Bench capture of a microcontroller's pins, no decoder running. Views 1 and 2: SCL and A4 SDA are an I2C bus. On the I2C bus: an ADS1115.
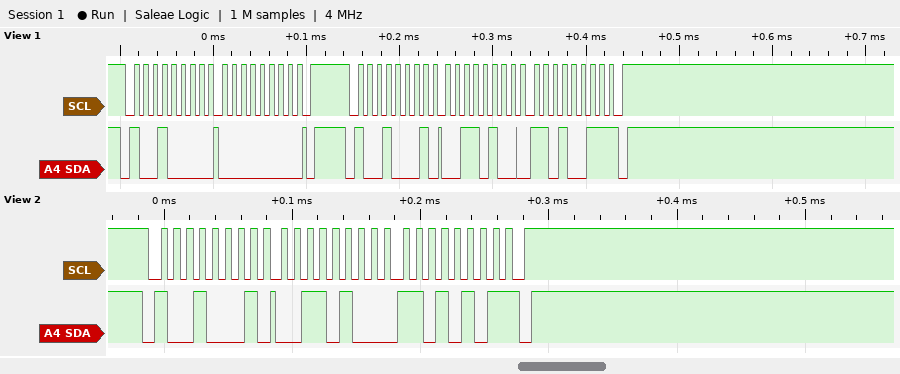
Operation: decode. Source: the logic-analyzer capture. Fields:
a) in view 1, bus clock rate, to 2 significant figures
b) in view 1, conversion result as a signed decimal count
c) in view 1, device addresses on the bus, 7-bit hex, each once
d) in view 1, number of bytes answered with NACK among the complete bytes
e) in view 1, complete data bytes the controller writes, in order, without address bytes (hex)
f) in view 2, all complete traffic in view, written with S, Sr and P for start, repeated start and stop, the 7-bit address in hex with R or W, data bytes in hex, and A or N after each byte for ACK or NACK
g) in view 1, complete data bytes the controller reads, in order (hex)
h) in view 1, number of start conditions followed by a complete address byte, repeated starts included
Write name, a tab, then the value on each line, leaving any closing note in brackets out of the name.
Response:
in view 1, bus clock rate, to 2 significant figures	100 kHz
in view 1, conversion result as a signed decimal count	13523
in view 1, device addresses on the bus, 7-bit hex, each once	0x48
in view 1, number of bytes answered with NACK among the complete bytes	1
in view 1, complete data bytes the controller writes, in order, without address bytes	00
in view 2, all complete traffic in view, written with S, Sr and P for start, repeated start and stop, the 7-bit address in hex with R or W, data bytes in hex, and A or N after each byte for ACK or NACK	S 48R A 34 A D5 N P
in view 1, complete data bytes the controller reads, in order	34 D3
in view 1, number of start conditions followed by a complete address byte, repeated starts included	2
